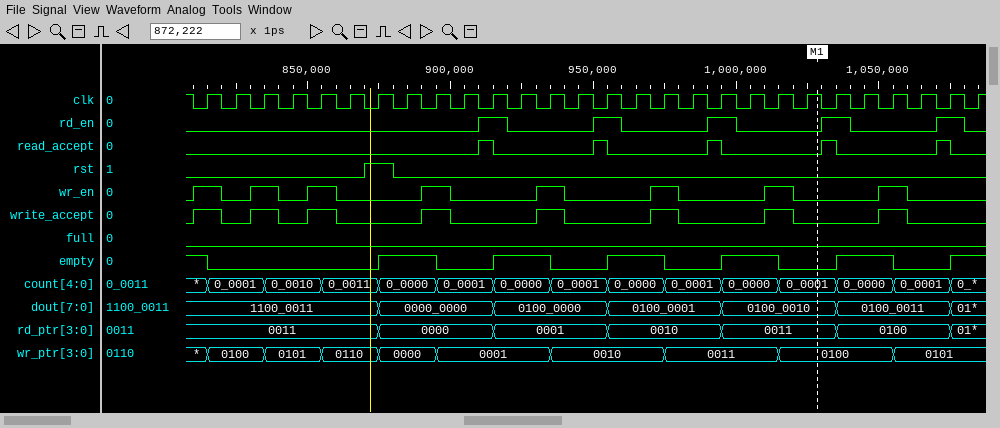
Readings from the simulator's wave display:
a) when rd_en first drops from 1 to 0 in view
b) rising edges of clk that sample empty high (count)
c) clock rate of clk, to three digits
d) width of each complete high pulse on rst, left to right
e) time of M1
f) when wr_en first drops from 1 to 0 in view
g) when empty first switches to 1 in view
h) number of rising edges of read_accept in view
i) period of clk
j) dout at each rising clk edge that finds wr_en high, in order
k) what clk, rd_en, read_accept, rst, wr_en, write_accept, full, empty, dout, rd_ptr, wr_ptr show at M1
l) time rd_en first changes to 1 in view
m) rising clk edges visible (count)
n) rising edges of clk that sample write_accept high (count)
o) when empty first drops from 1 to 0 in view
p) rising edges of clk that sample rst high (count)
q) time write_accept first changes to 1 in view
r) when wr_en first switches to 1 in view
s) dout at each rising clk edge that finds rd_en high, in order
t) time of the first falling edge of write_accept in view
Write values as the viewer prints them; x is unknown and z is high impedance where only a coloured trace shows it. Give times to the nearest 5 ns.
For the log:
920 ns
12
100 MHz
10 ns
1030 ns
820 ns
875 ns
5
10 ns
1100_0011, 1100_0011, 1100_0011, 0000_0000, 0100_0000, 0100_0001, 0100_0010, 0100_0011
clk=1, rd_en=0, read_accept=0, rst=0, wr_en=0, write_accept=0, full=0, empty=0, dout=0100_0010, rd_ptr=0011, wr_ptr=0100
910 ns
28
8
815 ns
1
810 ns
810 ns
0000_0000, 0100_0000, 0100_0001, 0100_0010, 0100_0011
820 ns
